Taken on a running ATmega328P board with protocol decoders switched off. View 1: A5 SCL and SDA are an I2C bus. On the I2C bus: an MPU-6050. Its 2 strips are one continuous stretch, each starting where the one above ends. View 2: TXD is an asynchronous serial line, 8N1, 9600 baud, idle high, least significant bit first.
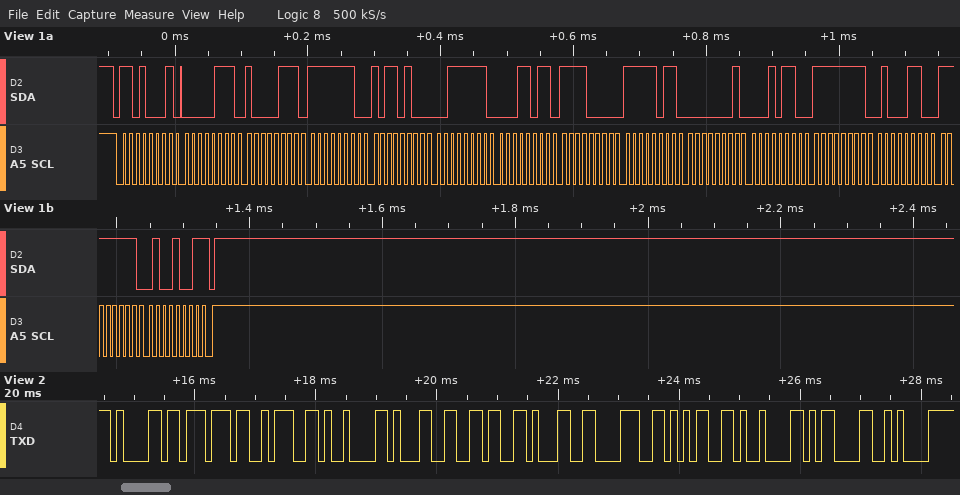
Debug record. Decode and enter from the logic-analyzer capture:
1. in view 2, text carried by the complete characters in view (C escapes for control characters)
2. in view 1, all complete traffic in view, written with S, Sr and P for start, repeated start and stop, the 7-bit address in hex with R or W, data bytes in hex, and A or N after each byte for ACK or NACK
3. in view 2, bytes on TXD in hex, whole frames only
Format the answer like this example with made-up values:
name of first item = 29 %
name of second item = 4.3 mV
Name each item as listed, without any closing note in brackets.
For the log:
in view 2, text carried by the complete characters in view = "aw:\t16185\t\r\n"
in view 1, all complete traffic in view, written with S, Sr and P for start, repeated start and stop, the 7-bit address in hex with R or W, data bytes in hex, and A or N after each byte for ACK or NACK = S 68R A 07 A 87 A FE A B4 A 3F A 1B A F0 A FB A 01 A 16 A FF A 46 A FF A 49 N P
in view 2, bytes on TXD in hex, whole frames only = 61 77 3A 09 31 36 31 38 35 09 0D 0A
